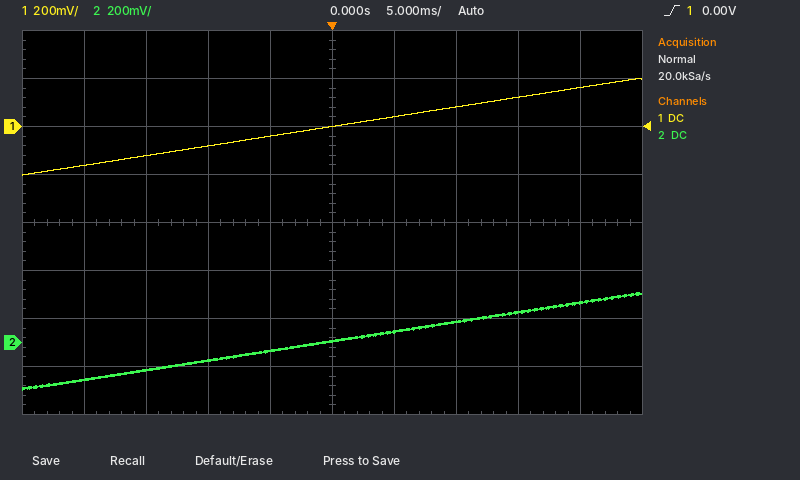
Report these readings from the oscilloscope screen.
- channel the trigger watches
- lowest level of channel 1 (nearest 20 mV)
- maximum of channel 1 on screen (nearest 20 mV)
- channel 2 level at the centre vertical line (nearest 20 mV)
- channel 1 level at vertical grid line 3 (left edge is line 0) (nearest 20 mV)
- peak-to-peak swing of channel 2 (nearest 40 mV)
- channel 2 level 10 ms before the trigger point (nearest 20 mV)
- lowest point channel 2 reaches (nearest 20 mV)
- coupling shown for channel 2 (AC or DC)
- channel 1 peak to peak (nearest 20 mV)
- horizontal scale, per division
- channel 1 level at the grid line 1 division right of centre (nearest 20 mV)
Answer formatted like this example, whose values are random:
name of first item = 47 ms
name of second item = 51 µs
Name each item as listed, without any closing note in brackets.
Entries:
channel the trigger watches = channel 1
lowest level of channel 1 = -200 mV
maximum of channel 1 on screen = 200 mV
channel 2 level at the centre vertical line = 0 mV
channel 1 level at vertical grid line 3 (left edge is line 0) = -80 mV
peak-to-peak swing of channel 2 = 400 mV
channel 2 level 10 ms before the trigger point = -80 mV
lowest point channel 2 reaches = -200 mV
coupling shown for channel 2 = DC
channel 1 peak to peak = 400 mV
horizontal scale, per division = 5 ms
channel 1 level at the grid line 1 division right of centre = 40 mV
